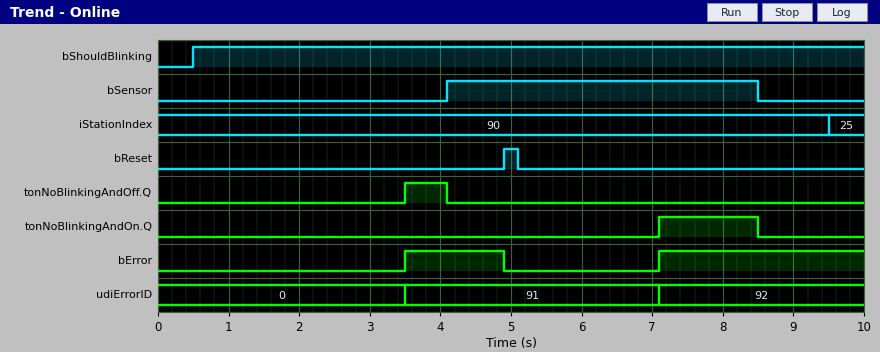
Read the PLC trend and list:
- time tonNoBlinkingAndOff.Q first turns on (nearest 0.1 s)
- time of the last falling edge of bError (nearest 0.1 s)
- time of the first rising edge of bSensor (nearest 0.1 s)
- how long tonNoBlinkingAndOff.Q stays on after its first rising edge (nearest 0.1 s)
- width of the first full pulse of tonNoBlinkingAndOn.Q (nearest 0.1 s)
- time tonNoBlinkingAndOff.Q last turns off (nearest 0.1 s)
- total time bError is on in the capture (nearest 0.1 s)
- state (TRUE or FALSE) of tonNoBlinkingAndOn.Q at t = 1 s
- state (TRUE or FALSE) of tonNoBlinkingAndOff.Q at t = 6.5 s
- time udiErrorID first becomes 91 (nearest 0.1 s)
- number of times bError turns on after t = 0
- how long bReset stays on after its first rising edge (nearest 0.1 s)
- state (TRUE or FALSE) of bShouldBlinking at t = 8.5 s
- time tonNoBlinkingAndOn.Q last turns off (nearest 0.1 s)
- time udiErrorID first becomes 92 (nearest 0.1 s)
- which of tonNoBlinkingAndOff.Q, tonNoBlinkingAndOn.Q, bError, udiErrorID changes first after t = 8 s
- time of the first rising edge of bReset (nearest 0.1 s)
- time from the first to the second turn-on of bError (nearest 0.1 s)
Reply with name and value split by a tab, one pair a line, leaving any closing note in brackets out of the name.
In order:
time tonNoBlinkingAndOff.Q first turns on	3.5 s
time of the last falling edge of bError	4.9 s
time of the first rising edge of bSensor	4.1 s
how long tonNoBlinkingAndOff.Q stays on after its first rising edge	0.6 s
width of the first full pulse of tonNoBlinkingAndOn.Q	1.4 s
time tonNoBlinkingAndOff.Q last turns off	4.1 s
total time bError is on in the capture	4.3 s
state (TRUE or FALSE) of tonNoBlinkingAndOn.Q at t = 1 s	FALSE
state (TRUE or FALSE) of tonNoBlinkingAndOff.Q at t = 6.5 s	FALSE
time udiErrorID first becomes 91	3.5 s
number of times bError turns on after t = 0	2
how long bReset stays on after its first rising edge	0.2 s
state (TRUE or FALSE) of bShouldBlinking at t = 8.5 s	TRUE
time tonNoBlinkingAndOn.Q last turns off	8.5 s
time udiErrorID first becomes 92	7.1 s
which of tonNoBlinkingAndOff.Q, tonNoBlinkingAndOn.Q, bError, udiErrorID changes first after t = 8 s	tonNoBlinkingAndOn.Q
time of the first rising edge of bReset	4.9 s
time from the first to the second turn-on of bError	3.6 s
